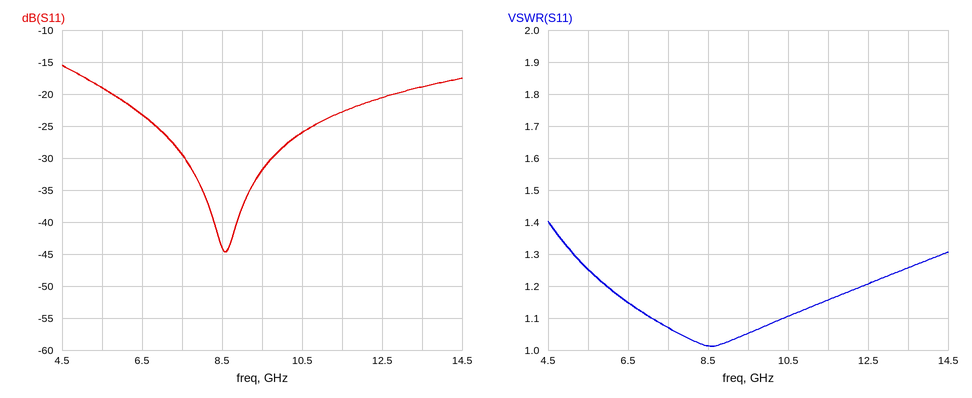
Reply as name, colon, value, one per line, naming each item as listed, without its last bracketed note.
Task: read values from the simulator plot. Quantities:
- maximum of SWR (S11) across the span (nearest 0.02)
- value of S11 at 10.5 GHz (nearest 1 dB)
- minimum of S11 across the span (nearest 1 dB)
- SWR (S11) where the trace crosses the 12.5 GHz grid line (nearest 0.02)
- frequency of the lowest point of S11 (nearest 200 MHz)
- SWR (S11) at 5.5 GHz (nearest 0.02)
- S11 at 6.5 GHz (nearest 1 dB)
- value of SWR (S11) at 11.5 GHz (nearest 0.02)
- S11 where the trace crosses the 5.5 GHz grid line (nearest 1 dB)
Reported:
maximum of SWR (S11) across the span: 1.40
value of S11 at 10.5 GHz: -26 dB
minimum of S11 across the span: -45 dB
SWR (S11) where the trace crosses the 12.5 GHz grid line: 1.20
frequency of the lowest point of S11: 8.6 GHz
SWR (S11) at 5.5 GHz: 1.26
S11 at 6.5 GHz: -23 dB
value of SWR (S11) at 11.5 GHz: 1.16
S11 where the trace crosses the 5.5 GHz grid line: -19 dB
